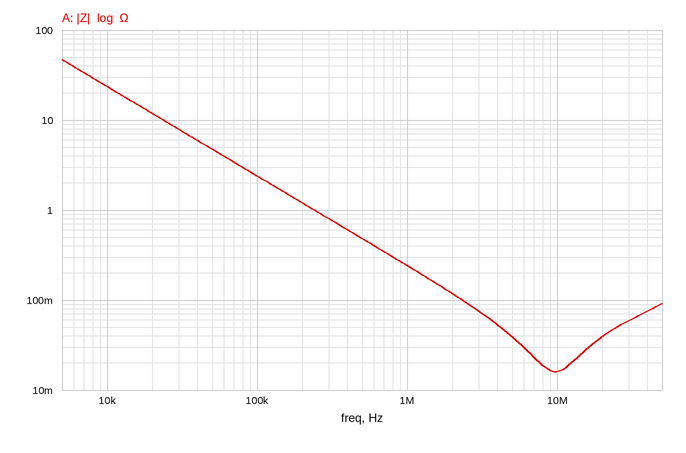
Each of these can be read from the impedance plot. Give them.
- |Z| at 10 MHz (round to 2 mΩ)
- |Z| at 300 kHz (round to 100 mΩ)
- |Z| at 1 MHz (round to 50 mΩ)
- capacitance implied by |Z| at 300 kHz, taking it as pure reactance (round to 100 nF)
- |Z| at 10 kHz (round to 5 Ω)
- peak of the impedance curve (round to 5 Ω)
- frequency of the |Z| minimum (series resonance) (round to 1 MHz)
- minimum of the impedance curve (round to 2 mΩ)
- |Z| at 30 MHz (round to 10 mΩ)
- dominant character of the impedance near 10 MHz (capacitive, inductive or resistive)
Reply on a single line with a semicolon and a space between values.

16 mΩ; 800 mΩ; 250 mΩ; 700 nF; 25 Ω; 45 Ω; 10 MHz; 16 mΩ; 60 mΩ; resistive
